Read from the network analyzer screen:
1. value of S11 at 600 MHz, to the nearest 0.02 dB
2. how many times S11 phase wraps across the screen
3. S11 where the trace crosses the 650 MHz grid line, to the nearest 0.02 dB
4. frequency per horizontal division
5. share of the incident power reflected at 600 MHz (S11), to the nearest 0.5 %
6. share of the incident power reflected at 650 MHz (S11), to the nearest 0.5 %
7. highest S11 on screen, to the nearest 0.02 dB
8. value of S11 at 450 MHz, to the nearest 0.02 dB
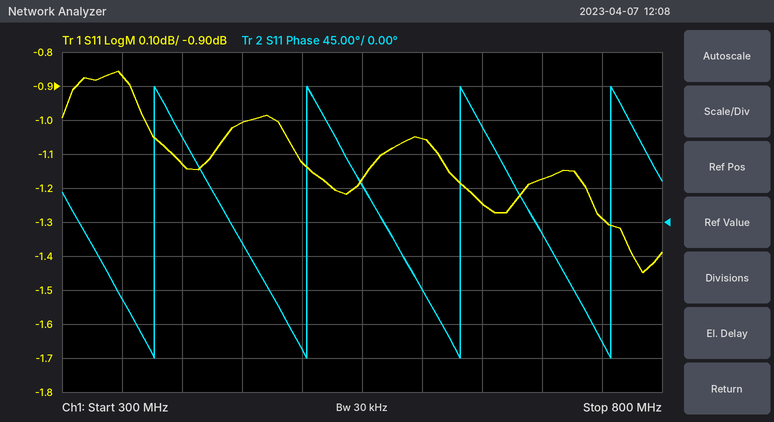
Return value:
-1.06 dB
4
-1.24 dB
50 MHz
78.5 %
75.0 %
-0.86 dB
-1.00 dB
